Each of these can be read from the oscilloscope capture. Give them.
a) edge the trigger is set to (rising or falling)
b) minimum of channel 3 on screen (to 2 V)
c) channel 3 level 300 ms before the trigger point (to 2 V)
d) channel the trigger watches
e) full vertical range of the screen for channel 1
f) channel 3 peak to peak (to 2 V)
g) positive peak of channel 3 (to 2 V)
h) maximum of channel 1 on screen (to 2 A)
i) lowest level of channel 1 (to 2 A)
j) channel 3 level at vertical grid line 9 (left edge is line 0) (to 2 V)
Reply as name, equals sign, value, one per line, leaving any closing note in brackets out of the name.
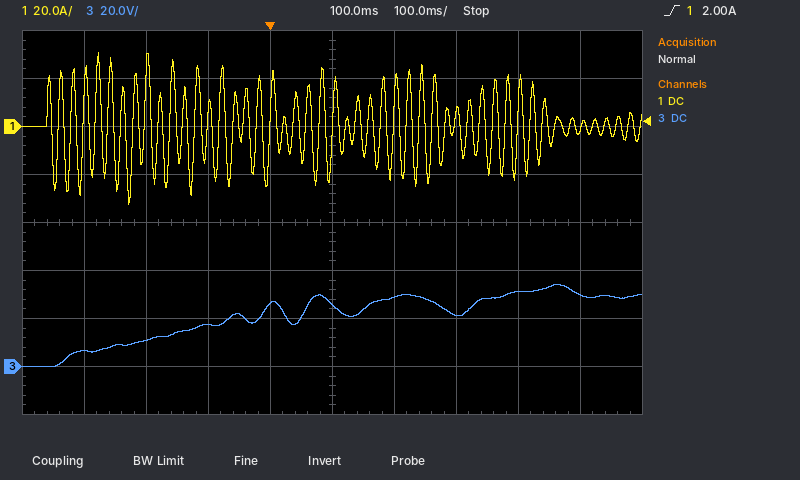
edge the trigger is set to = rising
minimum of channel 3 on screen = 0 V
channel 3 level 300 ms before the trigger point = 6 V
channel the trigger watches = channel 1
full vertical range of the screen for channel 1 = 160 A
channel 3 peak to peak = 34 V
positive peak of channel 3 = 34 V
maximum of channel 1 on screen = 30 A
lowest level of channel 1 = -32 A
channel 3 level at vertical grid line 9 (left edge is line 0) = 30 V
